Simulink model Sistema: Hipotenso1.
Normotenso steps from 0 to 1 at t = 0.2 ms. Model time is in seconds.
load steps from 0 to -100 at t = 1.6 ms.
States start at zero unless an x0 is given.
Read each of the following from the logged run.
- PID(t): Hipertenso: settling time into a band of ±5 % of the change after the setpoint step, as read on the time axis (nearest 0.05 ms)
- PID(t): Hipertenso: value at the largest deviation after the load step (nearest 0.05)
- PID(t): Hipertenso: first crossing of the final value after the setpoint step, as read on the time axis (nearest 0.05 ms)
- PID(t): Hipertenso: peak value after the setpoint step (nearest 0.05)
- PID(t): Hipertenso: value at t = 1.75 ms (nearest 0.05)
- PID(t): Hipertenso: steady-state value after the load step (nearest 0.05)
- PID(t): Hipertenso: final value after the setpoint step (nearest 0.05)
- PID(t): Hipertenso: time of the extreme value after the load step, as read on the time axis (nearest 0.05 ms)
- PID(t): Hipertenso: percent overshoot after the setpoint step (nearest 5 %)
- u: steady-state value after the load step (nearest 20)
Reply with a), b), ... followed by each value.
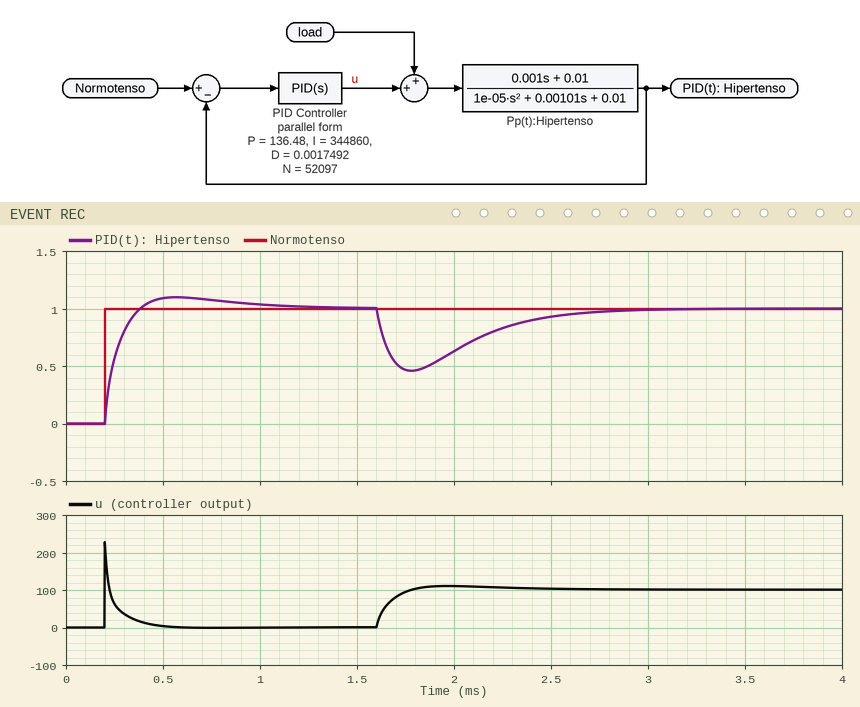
a) 0.90 ms
b) 0.45
c) 0.40 ms
d) 1.10
e) 0.45
f) 1.00
g) 1.00
h) 1.80 ms
i) 10 %
j) 100
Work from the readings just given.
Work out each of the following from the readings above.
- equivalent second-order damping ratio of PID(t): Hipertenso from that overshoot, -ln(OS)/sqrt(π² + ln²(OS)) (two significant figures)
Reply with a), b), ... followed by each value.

a) 0.59
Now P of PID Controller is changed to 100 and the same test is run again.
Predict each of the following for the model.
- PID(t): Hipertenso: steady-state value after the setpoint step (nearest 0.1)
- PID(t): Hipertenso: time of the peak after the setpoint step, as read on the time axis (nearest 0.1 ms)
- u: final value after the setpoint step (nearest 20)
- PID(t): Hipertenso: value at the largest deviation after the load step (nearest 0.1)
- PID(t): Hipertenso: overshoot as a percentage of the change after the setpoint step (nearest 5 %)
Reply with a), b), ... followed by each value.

a) 1.0
b) 0.6 ms
c) 0
d) 0.3
e) 15 %
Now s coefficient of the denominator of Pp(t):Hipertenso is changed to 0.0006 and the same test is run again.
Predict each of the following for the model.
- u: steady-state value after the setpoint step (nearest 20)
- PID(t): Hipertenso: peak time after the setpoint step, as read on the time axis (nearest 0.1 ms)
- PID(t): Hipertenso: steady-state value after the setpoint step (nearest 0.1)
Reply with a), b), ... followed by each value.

a) 0
b) 0.6 ms
c) 1.0
